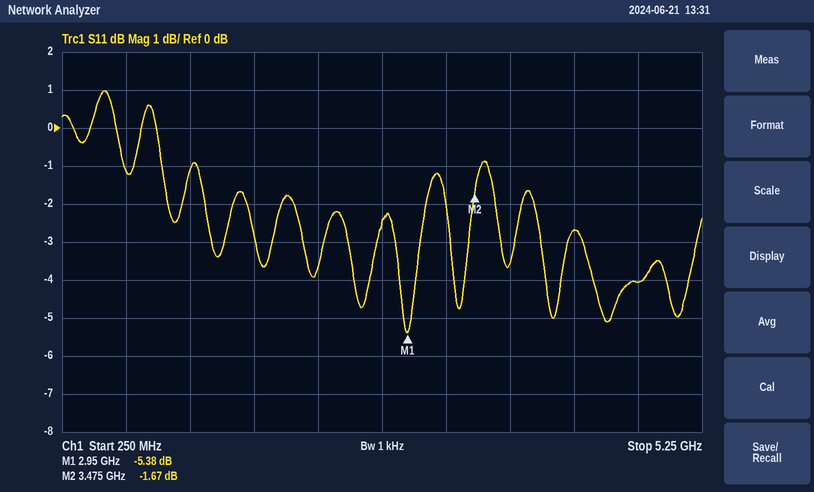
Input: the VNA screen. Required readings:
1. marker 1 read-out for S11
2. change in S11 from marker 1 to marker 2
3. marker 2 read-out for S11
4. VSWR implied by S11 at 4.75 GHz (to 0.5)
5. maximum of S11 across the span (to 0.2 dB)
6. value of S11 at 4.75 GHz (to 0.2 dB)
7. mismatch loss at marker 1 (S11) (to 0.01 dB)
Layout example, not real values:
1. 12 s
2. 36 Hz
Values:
1. -5.38 dB
2. 3.71 dB
3. -1.67 dB
4. 4.5
5. 1.0 dB
6. -4.0 dB
7. 1.49 dB
